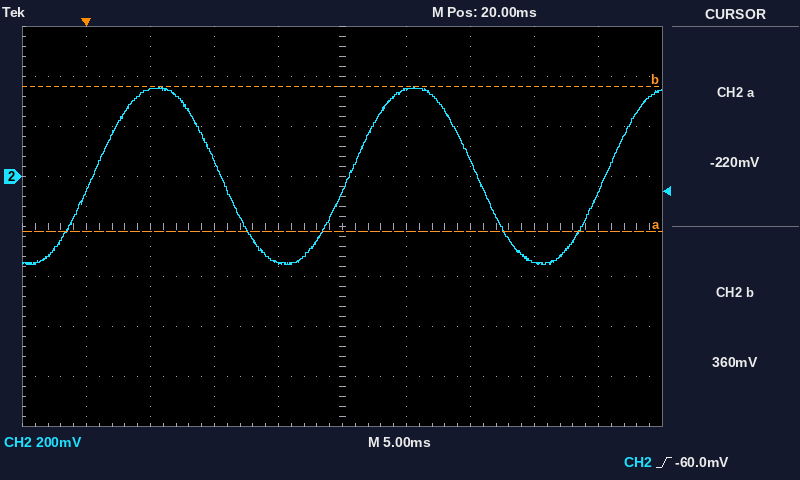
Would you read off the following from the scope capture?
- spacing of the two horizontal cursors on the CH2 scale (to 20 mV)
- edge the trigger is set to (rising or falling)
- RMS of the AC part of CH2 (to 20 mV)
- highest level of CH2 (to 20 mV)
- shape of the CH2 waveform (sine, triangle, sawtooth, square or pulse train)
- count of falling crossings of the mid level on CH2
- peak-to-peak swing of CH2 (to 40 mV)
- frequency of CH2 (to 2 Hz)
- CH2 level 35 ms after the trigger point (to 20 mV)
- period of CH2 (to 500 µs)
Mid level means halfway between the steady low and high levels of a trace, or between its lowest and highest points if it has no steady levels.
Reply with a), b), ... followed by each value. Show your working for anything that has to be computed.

a) 580 mV
b) rising
c) 720 mV / (2√2) ≈ 255 mV, so 260 mV to the nearest 20 mV
d) 360 mV
e) sine
f) 2
g) 720 mV
h) 1 / 20.0 ms ≈ 50 Hz
i) -340 mV
j) 20.0 ms
